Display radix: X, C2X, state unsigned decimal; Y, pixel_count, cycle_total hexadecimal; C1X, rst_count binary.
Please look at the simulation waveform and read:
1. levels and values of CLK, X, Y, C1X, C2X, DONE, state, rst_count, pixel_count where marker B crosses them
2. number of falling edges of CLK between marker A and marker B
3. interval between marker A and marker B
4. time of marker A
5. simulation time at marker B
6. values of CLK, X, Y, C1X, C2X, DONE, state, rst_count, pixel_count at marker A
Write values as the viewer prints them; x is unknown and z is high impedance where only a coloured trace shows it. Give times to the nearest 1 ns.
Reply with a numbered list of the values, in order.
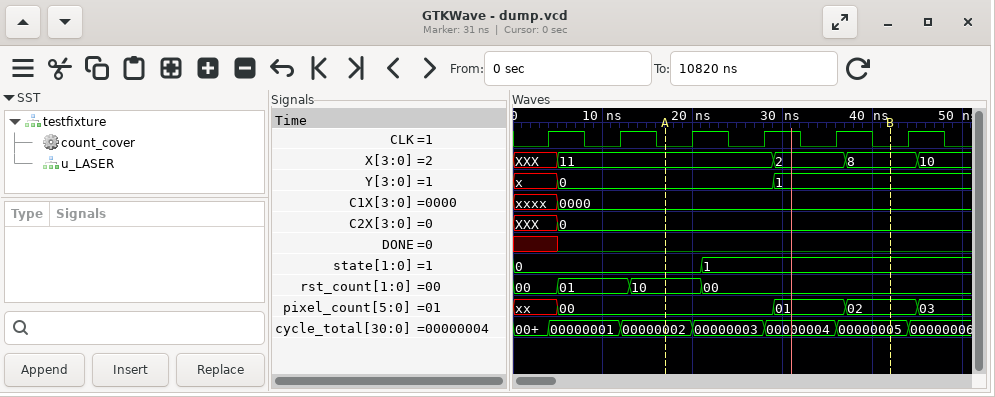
1. CLK=0, X=8, Y=1, C1X=0000, C2X=0, DONE=0, state=1, rst_count=00, pixel_count=02
2. 3
3. 25 ns
4. 17 ns
5. 42 ns
6. CLK=0, X=11, Y=0, C1X=0000, C2X=0, DONE=0, state=0, rst_count=10, pixel_count=00
